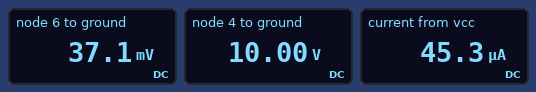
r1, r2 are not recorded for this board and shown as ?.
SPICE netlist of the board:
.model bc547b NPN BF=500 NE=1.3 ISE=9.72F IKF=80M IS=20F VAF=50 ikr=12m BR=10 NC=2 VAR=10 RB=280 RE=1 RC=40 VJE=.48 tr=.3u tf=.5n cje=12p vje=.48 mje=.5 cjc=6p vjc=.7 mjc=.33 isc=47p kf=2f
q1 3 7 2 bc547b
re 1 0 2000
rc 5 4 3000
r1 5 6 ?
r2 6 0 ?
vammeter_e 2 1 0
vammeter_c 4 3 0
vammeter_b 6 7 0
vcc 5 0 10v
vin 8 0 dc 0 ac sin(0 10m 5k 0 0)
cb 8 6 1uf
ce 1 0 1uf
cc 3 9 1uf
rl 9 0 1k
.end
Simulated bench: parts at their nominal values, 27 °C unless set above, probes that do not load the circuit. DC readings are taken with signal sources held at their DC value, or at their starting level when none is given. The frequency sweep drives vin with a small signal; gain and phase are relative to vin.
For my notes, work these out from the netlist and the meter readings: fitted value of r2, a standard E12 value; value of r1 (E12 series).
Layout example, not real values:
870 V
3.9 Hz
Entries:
820 Ω
220 kΩ
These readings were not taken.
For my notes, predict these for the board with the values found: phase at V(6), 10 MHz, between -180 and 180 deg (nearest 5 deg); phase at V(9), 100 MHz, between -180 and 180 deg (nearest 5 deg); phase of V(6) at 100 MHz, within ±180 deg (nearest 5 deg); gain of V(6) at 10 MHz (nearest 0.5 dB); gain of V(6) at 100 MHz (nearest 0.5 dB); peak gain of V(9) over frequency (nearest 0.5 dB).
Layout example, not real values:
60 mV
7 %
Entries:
0 deg
-25 deg
0 deg
0 dB
0 dB
-10.5 dB
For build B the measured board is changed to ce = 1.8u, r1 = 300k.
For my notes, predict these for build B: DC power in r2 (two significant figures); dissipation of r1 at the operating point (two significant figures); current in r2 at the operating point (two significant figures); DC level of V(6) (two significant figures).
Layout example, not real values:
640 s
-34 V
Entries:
910 nW
330 µW
33 µA
27 mV
